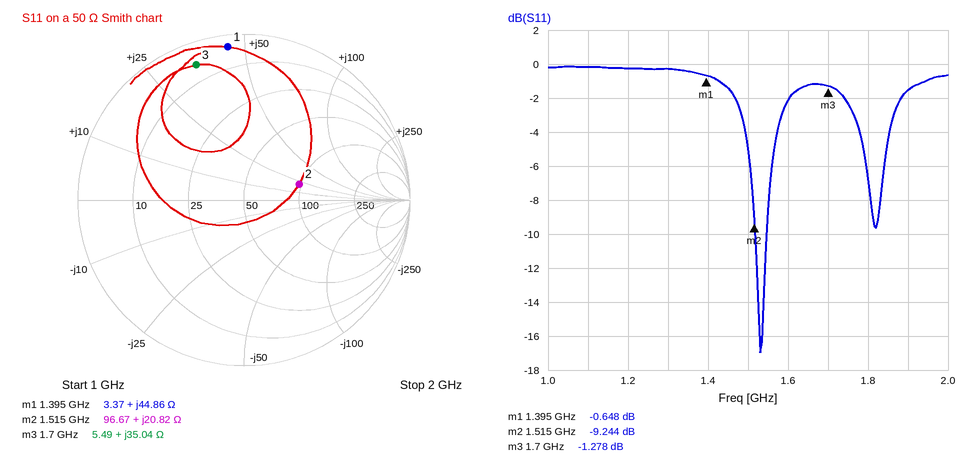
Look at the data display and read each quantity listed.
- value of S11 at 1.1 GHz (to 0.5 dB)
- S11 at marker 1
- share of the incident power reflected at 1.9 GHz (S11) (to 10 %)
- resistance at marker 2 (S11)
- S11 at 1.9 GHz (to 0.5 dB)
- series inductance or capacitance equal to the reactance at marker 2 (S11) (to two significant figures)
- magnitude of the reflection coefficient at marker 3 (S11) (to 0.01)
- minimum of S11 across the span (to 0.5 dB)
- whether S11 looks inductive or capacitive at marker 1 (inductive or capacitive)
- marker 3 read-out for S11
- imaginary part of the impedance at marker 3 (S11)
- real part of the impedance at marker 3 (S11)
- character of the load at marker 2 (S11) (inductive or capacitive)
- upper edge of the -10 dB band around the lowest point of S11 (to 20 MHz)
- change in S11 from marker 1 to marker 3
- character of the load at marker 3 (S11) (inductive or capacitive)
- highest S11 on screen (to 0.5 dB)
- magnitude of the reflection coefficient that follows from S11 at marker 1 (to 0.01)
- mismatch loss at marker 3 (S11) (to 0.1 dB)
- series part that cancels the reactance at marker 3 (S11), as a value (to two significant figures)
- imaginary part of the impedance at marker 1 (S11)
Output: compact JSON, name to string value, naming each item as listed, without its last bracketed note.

{"value of S11 at 1.1 GHz": "0.0 dB", "S11 at marker 1": "-0.648 dB", "share of the incident power reflected at 1.9 GHz (S11)": "70 %", "resistance at marker 2": "96.67 Ω", "S11 at 1.9 GHz": "-1.5 dB", "series inductance or capacitance equal to the reactance at marker 2 (S11)": "2.2 nH", "magnitude of the reflection coefficient at marker 3 (S11)": "0.86", "minimum of S11 across the span": "-17.0 dB", "whether S11 looks inductive or capacitive at marker 1": "inductive", "marker 3 read-out for S11": "-1.278 dB", "imaginary part of the impedance at marker 3": "+35.04 Ω", "real part of the impedance at marker 3": "5.49 Ω", "character of the load at marker 2 (S11)": "inductive", "upper edge of the -10 dB band around the lowest point of S11": "1.54 GHz", "change in S11 from marker 1 to marker 3": "-0.630 dB", "character of the load at marker 3 (S11)": "inductive", "highest S11 on screen": "0.0 dB", "magnitude of the reflection coefficient that follows from S11 at marker 1": "0.93", "mismatch loss at marker 3 (S11)": "5.9 dB", "series part that cancels the reactance at marker 3 (S11), as a value": "2.7 pF", "imaginary part of the impedance at marker 1": "+44.86 Ω"}
